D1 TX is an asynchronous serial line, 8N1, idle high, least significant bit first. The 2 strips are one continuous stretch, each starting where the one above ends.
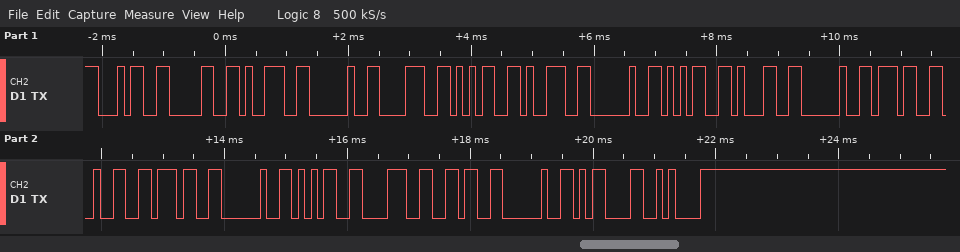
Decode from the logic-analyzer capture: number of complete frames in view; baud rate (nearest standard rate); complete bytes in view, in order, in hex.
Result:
21
9600 baud
0x34 0x30 0x39 0x20 0x38 0x35 0x39 0x20 0x35 0x31 0x20 0x37 0x32 0x37 0x20 0x35 0x38 0x36 0x20 0x0D 0x0A
